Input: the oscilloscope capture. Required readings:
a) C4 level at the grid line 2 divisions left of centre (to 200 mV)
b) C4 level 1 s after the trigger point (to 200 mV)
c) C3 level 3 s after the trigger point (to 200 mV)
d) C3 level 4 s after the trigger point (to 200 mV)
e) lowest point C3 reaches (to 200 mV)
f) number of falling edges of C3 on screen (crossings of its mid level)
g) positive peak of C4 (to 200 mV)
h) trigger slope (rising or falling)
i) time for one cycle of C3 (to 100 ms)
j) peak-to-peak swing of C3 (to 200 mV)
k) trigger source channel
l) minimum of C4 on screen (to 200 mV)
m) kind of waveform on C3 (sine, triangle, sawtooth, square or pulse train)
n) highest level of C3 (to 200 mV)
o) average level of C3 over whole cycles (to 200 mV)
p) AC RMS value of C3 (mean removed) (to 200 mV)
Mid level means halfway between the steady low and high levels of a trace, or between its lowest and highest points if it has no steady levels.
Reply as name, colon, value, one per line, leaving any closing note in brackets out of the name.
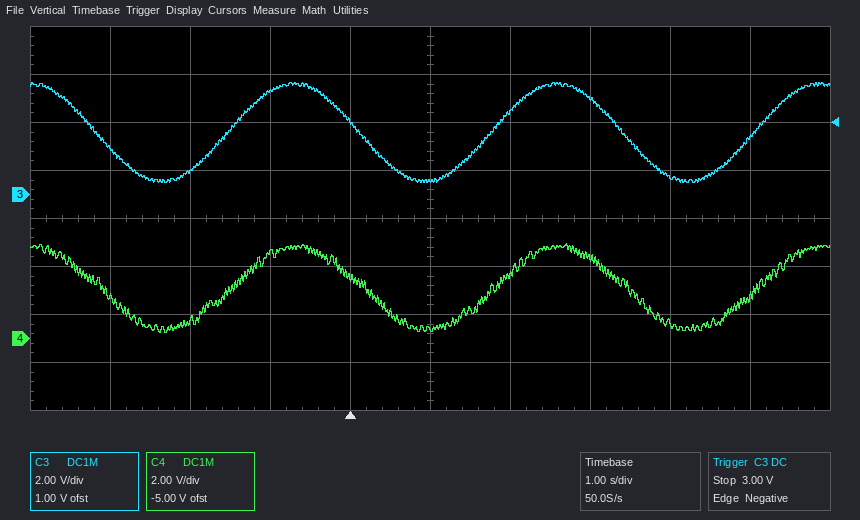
C4 level at the grid line 2 divisions left of centre: 3.6 V
C4 level 1 s after the trigger point: 400 mV
C3 level 3 s after the trigger point: 4.0 V
C3 level 4 s after the trigger point: 800 mV
lowest point C3 reaches: 400 mV
number of falling edges of C3 on screen: 3
positive peak of C4: 4.0 V
trigger slope: falling
time for one cycle of C3: 3.3 s
peak-to-peak swing of C3: 4.2 V
trigger source channel: C3
minimum of C4 on screen: 200 mV
kind of waveform on C3: sine
highest level of C3: 4.6 V
average level of C3 over whole cycles: 2.6 V
AC RMS value of C3 (mean removed): 1.4 V
